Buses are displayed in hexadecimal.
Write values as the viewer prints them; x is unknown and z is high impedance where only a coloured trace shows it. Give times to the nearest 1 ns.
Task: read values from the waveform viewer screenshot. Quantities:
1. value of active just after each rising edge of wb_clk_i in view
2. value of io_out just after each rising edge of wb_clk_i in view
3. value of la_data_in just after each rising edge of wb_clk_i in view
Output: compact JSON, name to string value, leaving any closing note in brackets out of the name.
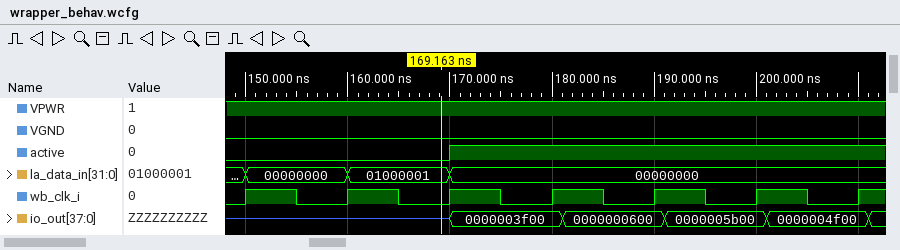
{"value of active just after each rising edge of wb_clk_i in view": "0 0 1 1 1 1 1", "value of io_out just after each rising edge of wb_clk_i in view": "z, z, 0000003f00, 0000003f00, 0000000600, 0000005b00, 0000004f00", "value of la_data_in just after each rising edge of wb_clk_i in view": "00000000, 01000001, 00000000, 00000000, 00000000, 00000000, 00000000"}
